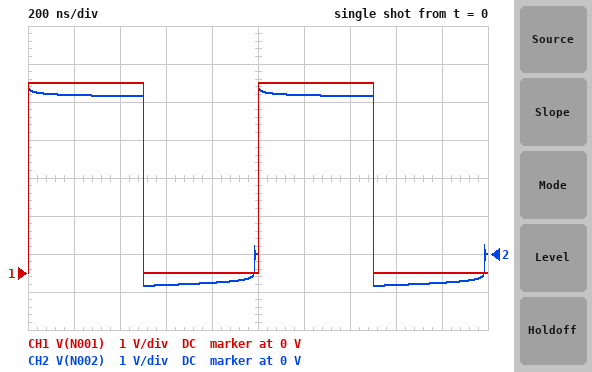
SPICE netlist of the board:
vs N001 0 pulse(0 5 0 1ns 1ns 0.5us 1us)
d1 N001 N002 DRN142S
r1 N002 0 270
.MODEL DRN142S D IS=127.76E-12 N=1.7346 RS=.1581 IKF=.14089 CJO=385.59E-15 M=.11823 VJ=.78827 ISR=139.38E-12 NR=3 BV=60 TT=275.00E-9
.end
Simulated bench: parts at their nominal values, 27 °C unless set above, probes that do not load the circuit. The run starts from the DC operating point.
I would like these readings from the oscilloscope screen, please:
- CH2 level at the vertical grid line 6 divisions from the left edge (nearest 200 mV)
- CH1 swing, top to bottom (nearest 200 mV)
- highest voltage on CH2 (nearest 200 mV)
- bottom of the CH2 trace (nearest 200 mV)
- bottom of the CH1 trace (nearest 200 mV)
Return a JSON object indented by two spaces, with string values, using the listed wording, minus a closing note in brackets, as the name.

{
  "CH2 level at the vertical grid line 6 divisions from the left edge": "4.2 V",
  "CH1 swing, top to bottom": "5.0 V",
  "highest voltage on CH2": "4.4 V",
  "bottom of the CH2 trace": "-800 mV",
  "bottom of the CH1 trace": "0 V"
}
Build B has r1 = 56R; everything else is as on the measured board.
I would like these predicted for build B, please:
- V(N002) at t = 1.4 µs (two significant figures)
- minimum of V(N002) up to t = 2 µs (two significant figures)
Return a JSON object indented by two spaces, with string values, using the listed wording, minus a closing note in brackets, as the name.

{
  "V(N002) at t = 1.4 µs": "4.1 V",
  "minimum of V(N002) up to t = 2 µs": "-920 mV"
}
